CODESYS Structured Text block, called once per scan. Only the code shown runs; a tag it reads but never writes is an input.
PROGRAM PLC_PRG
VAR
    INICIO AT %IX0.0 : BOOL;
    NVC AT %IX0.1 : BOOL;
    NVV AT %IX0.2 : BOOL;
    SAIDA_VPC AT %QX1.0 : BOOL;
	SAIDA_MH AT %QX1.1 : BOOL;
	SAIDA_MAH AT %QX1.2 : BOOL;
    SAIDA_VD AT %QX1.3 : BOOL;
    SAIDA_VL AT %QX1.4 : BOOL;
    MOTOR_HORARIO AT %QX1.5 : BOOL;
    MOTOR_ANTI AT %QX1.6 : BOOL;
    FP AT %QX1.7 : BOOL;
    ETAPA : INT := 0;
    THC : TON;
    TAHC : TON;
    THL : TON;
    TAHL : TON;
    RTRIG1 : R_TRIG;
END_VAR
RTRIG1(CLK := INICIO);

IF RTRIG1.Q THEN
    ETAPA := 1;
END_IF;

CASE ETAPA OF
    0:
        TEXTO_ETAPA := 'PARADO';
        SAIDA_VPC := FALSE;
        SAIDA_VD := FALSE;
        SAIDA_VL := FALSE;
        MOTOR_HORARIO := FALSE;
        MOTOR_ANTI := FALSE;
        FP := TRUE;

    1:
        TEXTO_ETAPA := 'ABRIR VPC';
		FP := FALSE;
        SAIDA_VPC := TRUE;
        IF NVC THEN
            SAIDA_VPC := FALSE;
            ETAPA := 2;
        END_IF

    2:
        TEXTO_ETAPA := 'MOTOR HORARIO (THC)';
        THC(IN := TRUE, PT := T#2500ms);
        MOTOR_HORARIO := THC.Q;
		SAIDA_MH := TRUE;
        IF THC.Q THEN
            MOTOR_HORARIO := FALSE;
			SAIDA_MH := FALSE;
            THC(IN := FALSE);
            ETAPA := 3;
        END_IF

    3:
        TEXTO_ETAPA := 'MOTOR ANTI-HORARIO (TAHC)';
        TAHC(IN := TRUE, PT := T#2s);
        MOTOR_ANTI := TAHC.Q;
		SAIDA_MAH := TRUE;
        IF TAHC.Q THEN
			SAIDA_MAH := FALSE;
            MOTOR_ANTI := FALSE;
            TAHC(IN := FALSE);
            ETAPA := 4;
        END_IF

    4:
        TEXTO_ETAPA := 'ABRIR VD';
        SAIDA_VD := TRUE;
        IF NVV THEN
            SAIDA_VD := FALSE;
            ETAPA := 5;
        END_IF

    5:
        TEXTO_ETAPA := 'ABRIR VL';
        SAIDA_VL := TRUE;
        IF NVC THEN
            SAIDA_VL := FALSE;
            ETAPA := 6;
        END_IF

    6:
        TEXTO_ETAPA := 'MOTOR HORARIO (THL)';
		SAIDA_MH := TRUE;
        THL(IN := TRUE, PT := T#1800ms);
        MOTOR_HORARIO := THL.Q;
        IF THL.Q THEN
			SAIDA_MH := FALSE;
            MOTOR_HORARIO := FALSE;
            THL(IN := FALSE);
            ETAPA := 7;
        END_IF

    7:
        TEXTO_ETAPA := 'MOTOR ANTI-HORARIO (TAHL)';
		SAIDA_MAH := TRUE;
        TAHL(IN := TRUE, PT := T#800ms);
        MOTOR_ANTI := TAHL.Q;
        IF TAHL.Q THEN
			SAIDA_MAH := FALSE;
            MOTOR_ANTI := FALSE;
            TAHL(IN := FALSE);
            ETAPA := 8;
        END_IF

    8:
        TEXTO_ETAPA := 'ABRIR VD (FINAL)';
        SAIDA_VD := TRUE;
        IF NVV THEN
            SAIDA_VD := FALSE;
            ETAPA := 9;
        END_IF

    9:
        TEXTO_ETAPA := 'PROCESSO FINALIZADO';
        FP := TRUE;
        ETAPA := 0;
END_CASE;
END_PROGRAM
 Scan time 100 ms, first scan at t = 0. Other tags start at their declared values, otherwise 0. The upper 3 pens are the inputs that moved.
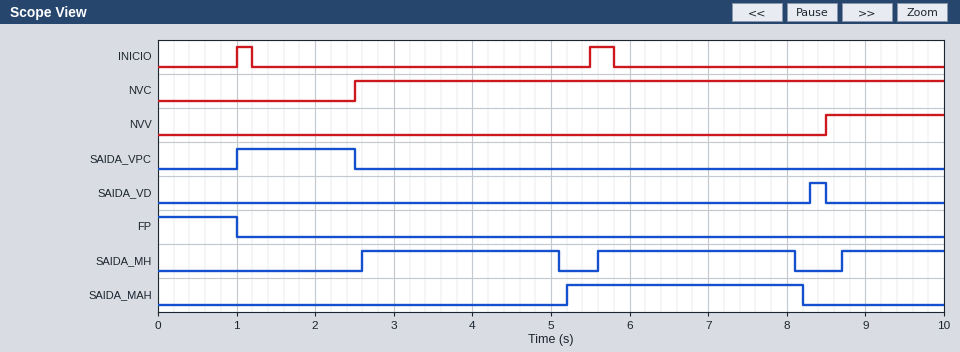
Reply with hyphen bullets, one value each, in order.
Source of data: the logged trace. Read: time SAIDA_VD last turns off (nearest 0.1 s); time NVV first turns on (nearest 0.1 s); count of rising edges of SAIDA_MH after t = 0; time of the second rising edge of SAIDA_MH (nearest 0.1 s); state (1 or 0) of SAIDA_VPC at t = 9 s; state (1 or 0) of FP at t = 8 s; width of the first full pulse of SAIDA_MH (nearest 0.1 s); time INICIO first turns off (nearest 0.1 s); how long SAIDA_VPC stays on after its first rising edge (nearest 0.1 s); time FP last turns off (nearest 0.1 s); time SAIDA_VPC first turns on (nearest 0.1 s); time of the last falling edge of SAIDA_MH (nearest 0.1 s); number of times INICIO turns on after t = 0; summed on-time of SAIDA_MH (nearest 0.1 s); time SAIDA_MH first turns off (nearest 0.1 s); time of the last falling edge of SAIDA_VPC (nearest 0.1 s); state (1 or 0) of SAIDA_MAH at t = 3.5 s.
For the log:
- 8.5 s
- 8.5 s
- 3
- 5.6 s
- 0
- 0
- 2.5 s
- 1.2 s
- 1.5 s
- 1.0 s
- 1.0 s
- 8.1 s
- 2
- 6.3 s
- 5.1 s
- 2.5 s
- 0
